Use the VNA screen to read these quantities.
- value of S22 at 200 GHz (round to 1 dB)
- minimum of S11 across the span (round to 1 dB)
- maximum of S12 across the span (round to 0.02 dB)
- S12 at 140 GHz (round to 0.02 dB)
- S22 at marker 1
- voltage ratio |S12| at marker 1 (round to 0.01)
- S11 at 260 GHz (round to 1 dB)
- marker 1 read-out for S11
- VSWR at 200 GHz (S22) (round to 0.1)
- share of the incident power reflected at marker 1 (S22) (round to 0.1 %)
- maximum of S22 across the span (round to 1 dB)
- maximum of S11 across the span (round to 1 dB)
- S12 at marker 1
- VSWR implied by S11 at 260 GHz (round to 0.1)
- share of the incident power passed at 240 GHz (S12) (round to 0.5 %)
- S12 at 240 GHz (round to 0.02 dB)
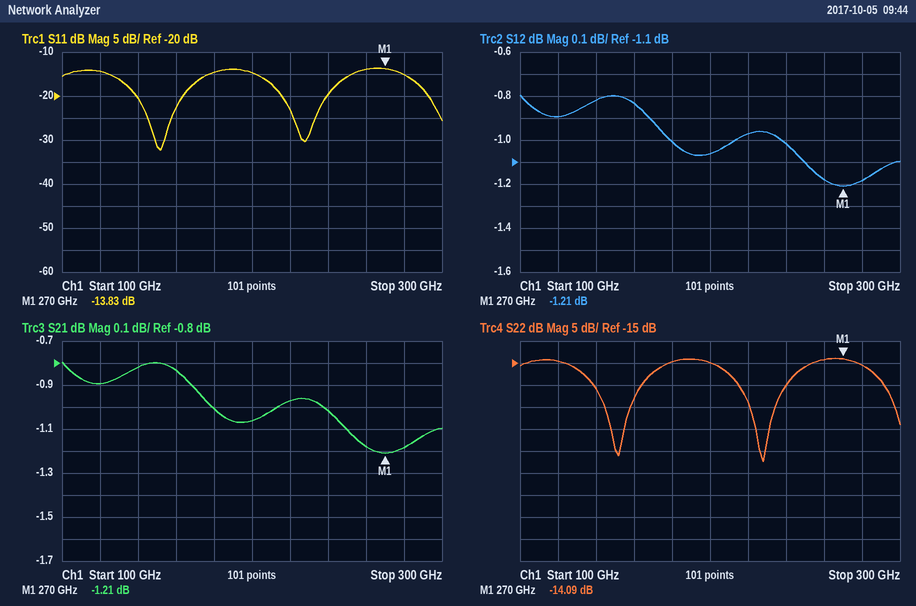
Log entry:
-15 dB
-32 dB
-0.80 dB
-0.82 dB
-14.09 dB
0.87
-14 dB
-13.83 dB
1.4
3.9 %
-14 dB
-14 dB
-1.21 dB
1.5
79.0 %
-1.02 dB
